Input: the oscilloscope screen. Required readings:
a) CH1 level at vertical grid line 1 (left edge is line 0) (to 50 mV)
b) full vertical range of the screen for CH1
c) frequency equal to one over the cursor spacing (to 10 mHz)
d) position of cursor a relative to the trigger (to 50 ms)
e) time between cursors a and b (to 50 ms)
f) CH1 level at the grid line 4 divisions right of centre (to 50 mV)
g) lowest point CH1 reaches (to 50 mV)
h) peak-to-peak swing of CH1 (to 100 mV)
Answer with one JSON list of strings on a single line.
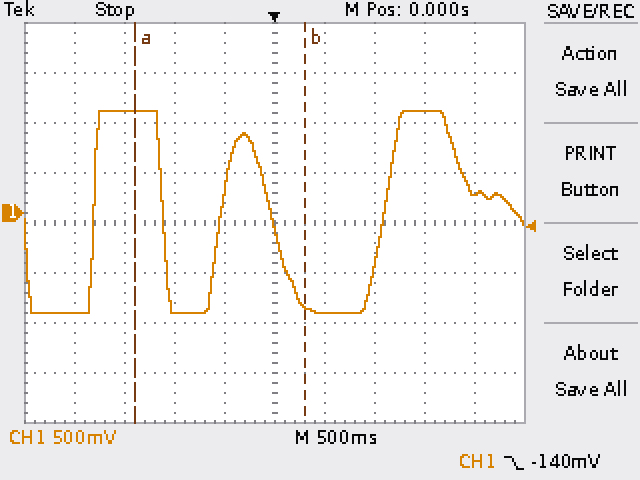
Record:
["-1.00 V", "4 V", "590 mHz", "-1.40 s", "1.70 s", "200 mV", "-1.00 V", "2.00 V"]
